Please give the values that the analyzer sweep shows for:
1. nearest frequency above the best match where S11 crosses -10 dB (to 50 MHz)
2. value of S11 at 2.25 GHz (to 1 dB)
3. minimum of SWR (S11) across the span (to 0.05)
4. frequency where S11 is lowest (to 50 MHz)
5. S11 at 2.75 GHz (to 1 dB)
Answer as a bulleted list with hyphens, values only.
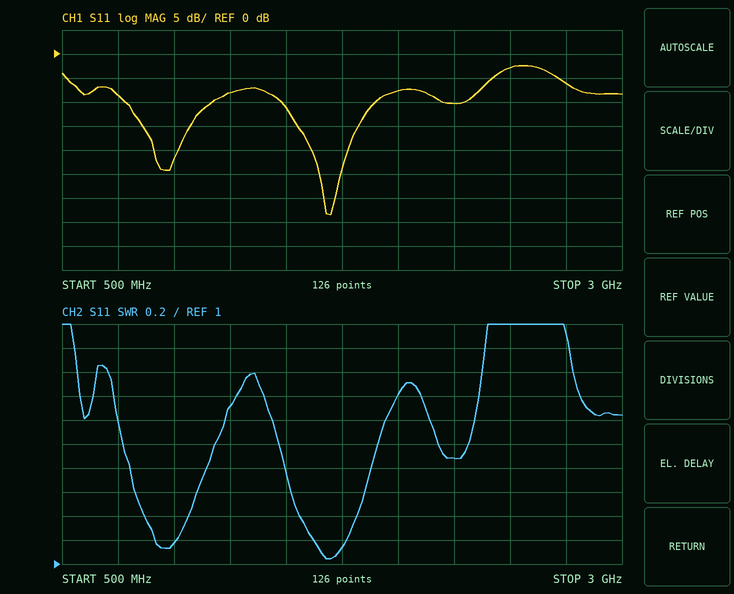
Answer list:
- 1.90 GHz
- -10 dB
- 1.05
- 1.70 GHz
- -6 dB
